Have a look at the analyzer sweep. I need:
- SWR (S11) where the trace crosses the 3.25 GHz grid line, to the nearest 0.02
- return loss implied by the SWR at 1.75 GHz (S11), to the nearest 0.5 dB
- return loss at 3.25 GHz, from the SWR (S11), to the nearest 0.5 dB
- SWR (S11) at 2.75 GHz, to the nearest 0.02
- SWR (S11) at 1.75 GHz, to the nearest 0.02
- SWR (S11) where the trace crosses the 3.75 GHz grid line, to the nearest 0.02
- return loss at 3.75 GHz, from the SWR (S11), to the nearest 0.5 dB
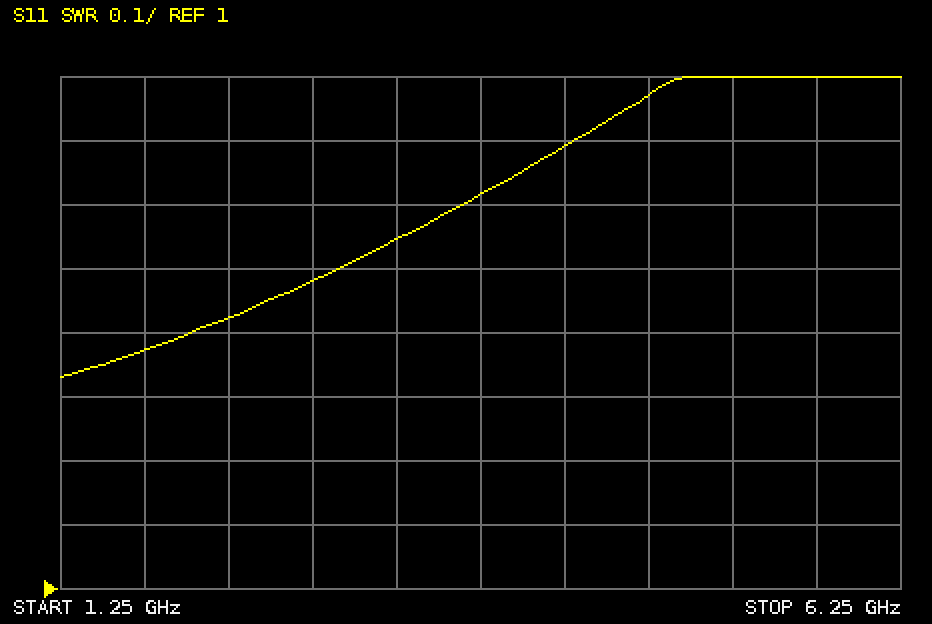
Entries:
1.54
16.0 dB
13.5 dB
1.48
1.38
1.62
12.5 dB
